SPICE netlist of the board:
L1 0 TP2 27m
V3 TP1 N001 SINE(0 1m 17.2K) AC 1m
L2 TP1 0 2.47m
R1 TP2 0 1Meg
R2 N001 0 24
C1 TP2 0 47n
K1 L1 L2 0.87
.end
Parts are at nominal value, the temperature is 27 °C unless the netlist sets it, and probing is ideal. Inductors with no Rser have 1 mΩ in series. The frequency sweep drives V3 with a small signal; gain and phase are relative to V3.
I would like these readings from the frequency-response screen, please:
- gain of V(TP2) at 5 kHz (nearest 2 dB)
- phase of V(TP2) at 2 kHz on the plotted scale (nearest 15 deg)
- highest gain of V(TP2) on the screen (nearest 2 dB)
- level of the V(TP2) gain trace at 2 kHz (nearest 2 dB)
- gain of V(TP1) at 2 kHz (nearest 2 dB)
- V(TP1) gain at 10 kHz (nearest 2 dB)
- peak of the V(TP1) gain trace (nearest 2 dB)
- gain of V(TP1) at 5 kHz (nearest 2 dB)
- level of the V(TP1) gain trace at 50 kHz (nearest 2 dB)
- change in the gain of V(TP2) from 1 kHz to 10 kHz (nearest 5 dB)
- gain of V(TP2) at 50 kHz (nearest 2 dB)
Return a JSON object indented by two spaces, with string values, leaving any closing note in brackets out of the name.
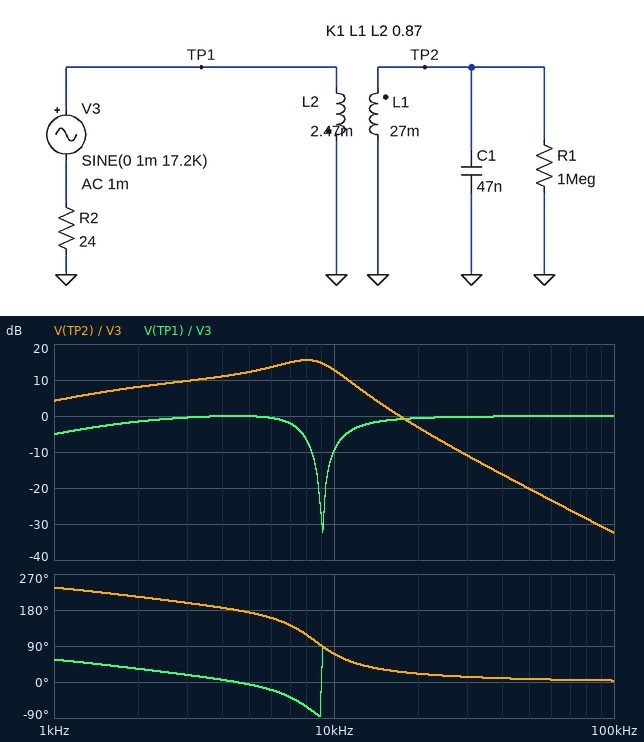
{
  "gain of V(TP2) at 5 kHz": "12 dB",
  "phase of V(TP2) at 2 kHz on the plotted scale": "210 deg",
  "highest gain of V(TP2) on the screen": "16 dB",
  "level of the V(TP2) gain trace at 2 kHz": "8 dB",
  "gain of V(TP1) at 2 kHz": "-2 dB",
  "V(TP1) gain at 10 kHz": "-10 dB",
  "peak of the V(TP1) gain trace": "0 dB",
  "gain of V(TP1) at 5 kHz": "0 dB",
  "level of the V(TP1) gain trace at 50 kHz": "0 dB",
  "change in the gain of V(TP2) from 1 kHz to 10 kHz": "10 dB",
  "gain of V(TP2) at 50 kHz": "-20 dB"
}
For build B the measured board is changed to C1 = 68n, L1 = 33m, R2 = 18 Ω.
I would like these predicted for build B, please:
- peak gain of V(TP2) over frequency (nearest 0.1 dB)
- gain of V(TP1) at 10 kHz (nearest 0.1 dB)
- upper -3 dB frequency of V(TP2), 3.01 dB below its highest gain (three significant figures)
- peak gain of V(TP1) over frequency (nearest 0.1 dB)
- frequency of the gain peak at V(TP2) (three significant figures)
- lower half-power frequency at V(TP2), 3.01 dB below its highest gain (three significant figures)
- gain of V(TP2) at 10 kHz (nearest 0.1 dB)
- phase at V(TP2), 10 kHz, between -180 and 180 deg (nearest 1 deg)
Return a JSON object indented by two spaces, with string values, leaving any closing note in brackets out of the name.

{
  "peak gain of V(TP2) over frequency": "16.4 dB",
  "gain of V(TP1) at 10 kHz": "-2.1 dB",
  "upper -3 dB frequency of V(TP2), 3.01 dB below its highest gain": "7.62 kHz",
  "peak gain of V(TP1) over frequency": "0 dB",
  "frequency of the gain peak at V(TP2)": "6.01 kHz",
  "lower half-power frequency at V(TP2), 3.01 dB below its highest gain": "3.92 kHz",
  "gain of V(TP2) at 10 kHz": "6.7 dB",
  "phase at V(TP2), 10 kHz, between -180 and 180 deg": "38 deg"
}
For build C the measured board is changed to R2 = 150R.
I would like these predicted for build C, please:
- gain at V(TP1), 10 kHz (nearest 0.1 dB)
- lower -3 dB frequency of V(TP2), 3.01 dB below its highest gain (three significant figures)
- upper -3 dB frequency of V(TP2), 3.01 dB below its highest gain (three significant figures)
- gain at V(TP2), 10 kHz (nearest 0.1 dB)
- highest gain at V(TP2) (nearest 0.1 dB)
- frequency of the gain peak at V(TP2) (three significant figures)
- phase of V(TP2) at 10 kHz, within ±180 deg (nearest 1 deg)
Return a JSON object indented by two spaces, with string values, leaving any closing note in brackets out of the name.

{
  "gain at V(TP1), 10 kHz": "-25.0 dB",
  "lower -3 dB frequency of V(TP2), 3.01 dB below its highest gain": "3.82 kHz",
  "upper -3 dB frequency of V(TP2), 3.01 dB below its highest gain": "5.43 kHz",
  "gain at V(TP2), 10 kHz": "-2.6 dB",
  "highest gain at V(TP2)": "11.6 dB",
  "frequency of the gain peak at V(TP2)": "4.56 kHz",
  "phase of V(TP2) at 10 kHz, within ±180 deg": "87 deg"
}
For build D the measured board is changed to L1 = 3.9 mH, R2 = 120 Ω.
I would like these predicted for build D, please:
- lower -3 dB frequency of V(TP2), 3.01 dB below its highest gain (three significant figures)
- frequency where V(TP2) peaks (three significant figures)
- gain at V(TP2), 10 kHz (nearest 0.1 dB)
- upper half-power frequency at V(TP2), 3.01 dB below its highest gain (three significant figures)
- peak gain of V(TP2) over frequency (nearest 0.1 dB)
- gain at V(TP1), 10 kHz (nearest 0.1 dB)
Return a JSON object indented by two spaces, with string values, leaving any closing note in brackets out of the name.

{
  "lower -3 dB frequency of V(TP2), 3.01 dB below its highest gain": "8.56 kHz",
  "frequency where V(TP2) peaks": "15.4 kHz",
  "gain at V(TP2), 10 kHz": "2.2 dB",
  "upper half-power frequency at V(TP2), 3.01 dB below its highest gain": "23.2 kHz",
  "peak gain of V(TP2) over frequency": "4.1 dB",
  "gain at V(TP1), 10 kHz": "-0.3 dB"
}
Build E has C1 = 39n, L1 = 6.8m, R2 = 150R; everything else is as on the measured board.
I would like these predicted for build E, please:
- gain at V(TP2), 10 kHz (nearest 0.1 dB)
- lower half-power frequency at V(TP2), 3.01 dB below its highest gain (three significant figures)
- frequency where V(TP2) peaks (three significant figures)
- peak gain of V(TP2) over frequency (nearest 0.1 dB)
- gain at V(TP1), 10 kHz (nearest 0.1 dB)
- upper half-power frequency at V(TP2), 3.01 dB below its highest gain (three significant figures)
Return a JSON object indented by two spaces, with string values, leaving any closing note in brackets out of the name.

{
  "gain at V(TP2), 10 kHz": "5.7 dB",
  "lower half-power frequency at V(TP2), 3.01 dB below its highest gain": "7.36 kHz",
  "frequency where V(TP2) peaks": "10.9 kHz",
  "peak gain of V(TP2) over frequency": "5.9 dB",
  "gain at V(TP1), 10 kHz": "0 dB",
  "upper half-power frequency at V(TP2), 3.01 dB below its highest gain": "15.6 kHz"
}
